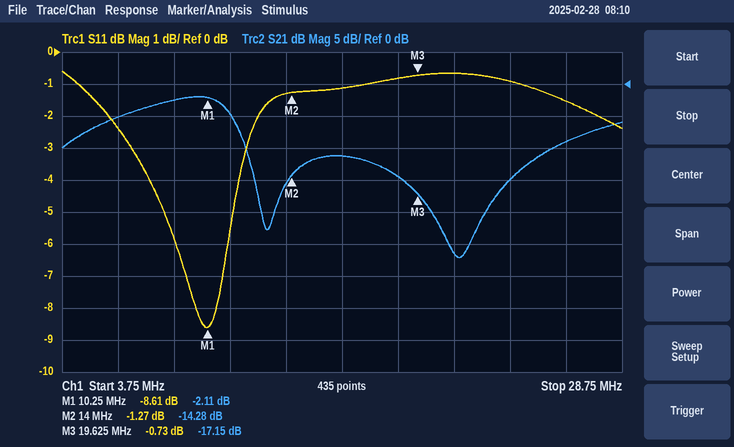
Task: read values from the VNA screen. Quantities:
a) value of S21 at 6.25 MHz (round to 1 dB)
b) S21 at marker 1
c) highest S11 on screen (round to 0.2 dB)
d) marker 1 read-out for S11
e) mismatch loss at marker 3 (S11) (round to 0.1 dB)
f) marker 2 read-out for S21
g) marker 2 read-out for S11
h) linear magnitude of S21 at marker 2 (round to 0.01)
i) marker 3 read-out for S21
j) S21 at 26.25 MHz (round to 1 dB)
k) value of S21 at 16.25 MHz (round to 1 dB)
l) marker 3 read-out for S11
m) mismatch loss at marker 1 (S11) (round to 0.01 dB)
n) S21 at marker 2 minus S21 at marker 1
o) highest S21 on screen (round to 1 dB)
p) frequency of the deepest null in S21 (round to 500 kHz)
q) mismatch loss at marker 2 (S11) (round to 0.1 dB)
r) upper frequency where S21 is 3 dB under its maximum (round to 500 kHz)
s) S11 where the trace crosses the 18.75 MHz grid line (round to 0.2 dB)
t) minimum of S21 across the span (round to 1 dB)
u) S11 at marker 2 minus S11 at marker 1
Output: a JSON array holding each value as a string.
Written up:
["-5 dB", "-2.11 dB", "-0.6 dB", "-8.61 dB", "8.1 dB", "-14.28 dB", "-1.27 dB", "0.19", "-17.15 dB", "-9 dB", "-11 dB", "-0.73 dB", "0.64 dB", "-12.17 dB", "-2 dB", "21.5 MHz", "6.0 dB", "11.5 MHz", "-0.8 dB", "-27 dB", "7.34 dB"]
